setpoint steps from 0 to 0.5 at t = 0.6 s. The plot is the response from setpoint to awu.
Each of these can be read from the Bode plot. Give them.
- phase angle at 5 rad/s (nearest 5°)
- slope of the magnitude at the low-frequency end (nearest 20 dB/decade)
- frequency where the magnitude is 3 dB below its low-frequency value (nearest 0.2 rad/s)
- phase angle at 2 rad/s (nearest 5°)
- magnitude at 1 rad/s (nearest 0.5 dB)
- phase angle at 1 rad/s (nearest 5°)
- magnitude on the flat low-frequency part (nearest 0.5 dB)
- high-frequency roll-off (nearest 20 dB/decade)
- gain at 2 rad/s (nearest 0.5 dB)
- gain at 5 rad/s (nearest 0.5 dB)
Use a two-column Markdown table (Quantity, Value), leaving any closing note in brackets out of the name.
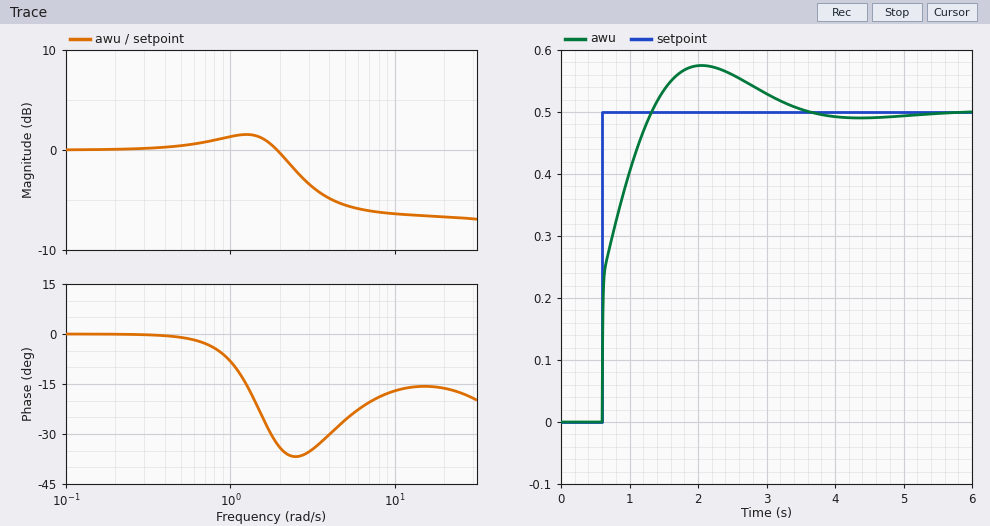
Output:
| Quantity | Value |
|---|---|
| phase angle at 5 rad/s | -25° |
| slope of the magnitude at the low-frequency end | 0 dB/decade |
| frequency where the magnitude is 3 dB below its low-frequency value | 2.8 rad/s |
| phase angle at 2 rad/s | -35° |
| magnitude at 1 rad/s | 1.5 dB |
| phase angle at 1 rad/s | -10° |
| magnitude on the flat low-frequency part | 0.0 dB |
| high-frequency roll-off | 0 dB/decade |
| gain at 2 rad/s | -0.5 dB |
| gain at 5 rad/s | -5.5 dB |
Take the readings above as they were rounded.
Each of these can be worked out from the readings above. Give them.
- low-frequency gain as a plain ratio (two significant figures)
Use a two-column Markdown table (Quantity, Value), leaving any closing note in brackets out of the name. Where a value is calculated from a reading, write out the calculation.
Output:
| Quantity | Value |
|---|---|
| low-frequency gain as a plain ratio | 10^(0 / 20) = 1.0 |
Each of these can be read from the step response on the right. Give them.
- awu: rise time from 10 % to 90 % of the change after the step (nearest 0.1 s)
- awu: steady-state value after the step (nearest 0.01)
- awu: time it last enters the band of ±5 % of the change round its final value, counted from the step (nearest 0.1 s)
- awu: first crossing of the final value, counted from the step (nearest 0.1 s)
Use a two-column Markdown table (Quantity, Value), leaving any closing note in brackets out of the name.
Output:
| Quantity | Value |
|---|---|
| awu: rise time from 10 % to 90 % of the change after the step | 0.5 s |
| awu: steady-state value after the step | 0.50 |
| awu: time it last enters the band of ±5 % of the change round its final value, counted from the step | 2.5 s |
| awu: first crossing of the final value, counted from the step | 0.7 s |
